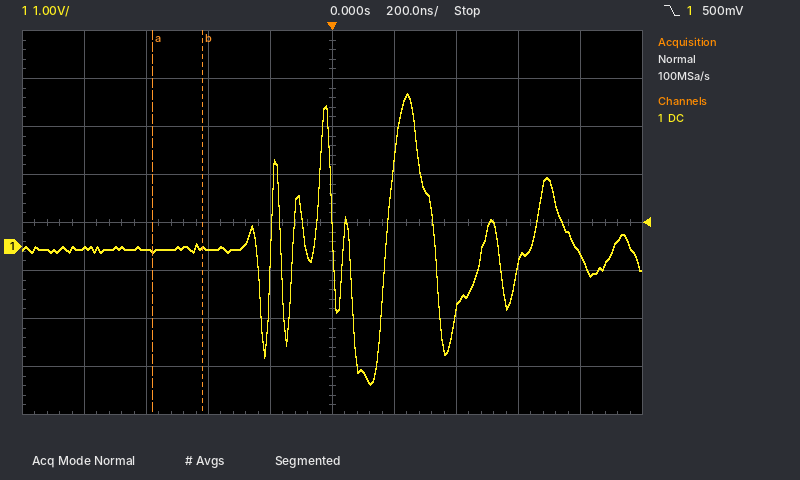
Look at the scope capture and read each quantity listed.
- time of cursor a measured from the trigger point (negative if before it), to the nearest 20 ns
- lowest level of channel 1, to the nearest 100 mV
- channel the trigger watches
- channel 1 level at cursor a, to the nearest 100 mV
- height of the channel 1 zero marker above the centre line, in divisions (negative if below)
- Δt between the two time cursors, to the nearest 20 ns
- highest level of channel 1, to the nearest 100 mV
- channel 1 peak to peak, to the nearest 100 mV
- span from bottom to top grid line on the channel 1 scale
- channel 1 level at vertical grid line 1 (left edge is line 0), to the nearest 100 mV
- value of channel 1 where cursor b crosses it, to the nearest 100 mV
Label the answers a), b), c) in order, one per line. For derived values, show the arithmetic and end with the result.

a) -580 ns
b) -2.9 V
c) channel 1
d) -100 mV
e) -0.5 div
f) 160 ns
g) 3.2 V
h) 3.2 V − (-2.9 V) = 6.1 V
i) 8 V
j) 0.0 V
k) 0.0 V
